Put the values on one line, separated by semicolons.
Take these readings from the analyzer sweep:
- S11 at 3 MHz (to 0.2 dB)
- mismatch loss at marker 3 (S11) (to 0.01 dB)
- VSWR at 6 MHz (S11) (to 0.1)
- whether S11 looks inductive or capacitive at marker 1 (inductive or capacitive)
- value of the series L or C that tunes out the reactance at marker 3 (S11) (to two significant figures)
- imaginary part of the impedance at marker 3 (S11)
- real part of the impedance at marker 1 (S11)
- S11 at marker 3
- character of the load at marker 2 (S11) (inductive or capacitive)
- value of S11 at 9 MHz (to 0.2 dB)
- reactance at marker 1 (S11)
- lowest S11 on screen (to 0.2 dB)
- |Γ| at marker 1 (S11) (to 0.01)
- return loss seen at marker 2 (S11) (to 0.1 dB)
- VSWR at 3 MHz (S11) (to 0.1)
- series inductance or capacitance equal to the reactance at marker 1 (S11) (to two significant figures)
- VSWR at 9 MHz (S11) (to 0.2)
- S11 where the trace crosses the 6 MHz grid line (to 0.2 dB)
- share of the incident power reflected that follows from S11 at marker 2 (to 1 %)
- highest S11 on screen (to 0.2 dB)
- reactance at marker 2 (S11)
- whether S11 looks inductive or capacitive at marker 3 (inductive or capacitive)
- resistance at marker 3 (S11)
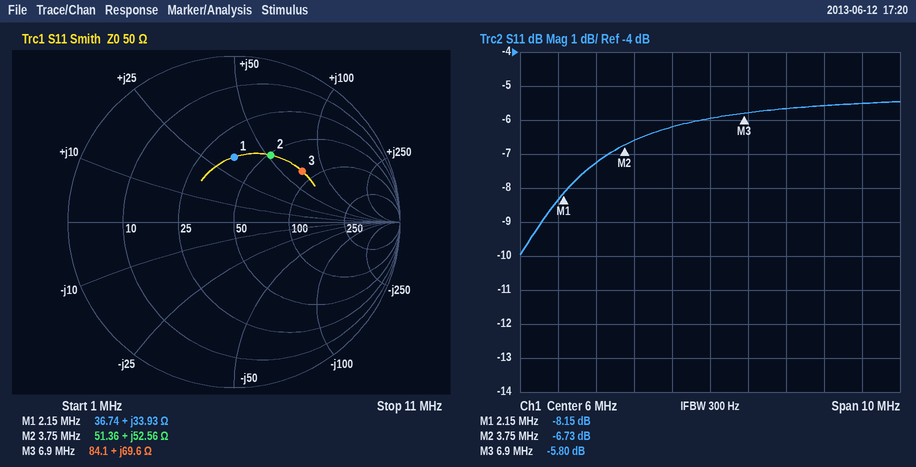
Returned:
-7.2 dB; 1.33 dB; 3.0; inductive; 330 pF; +69.6 Ω; 36.74 Ω; -5.80 dB; inductive; -5.6 dB; +33.93 Ω; -10.0 dB; 0.39; 6.7 dB; 2.5; 2.5 µH; 3.2; -6.0 dB; 21 %; -5.4 dB; +52.56 Ω; inductive; 84.1 Ω
